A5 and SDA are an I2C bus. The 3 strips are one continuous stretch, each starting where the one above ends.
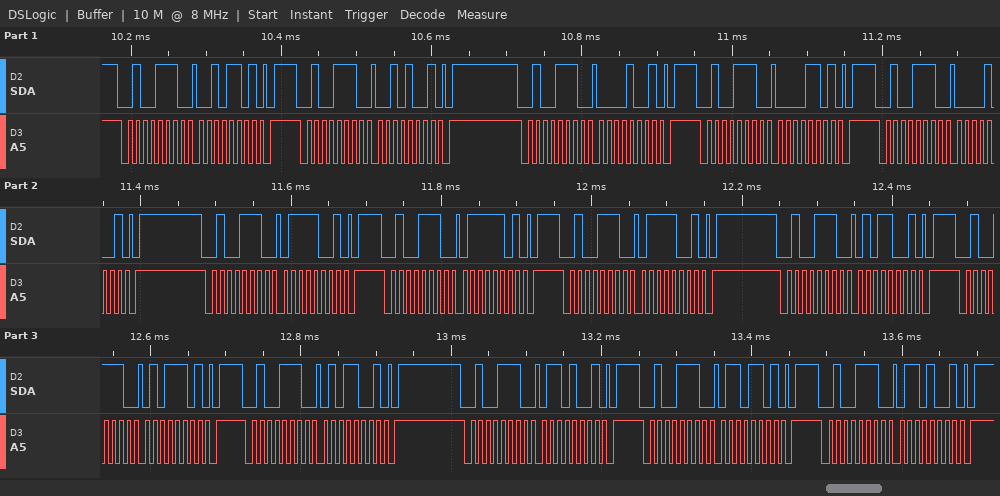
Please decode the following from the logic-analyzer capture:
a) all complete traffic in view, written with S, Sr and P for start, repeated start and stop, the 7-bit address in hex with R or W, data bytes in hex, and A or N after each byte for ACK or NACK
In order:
S 27W A 2D A P S 27W A 29 A P S 27W A 09 A P S 27W A 0D A P S 27W A 09 A P S 27W A 79 A P S 27W A 7D A P S 27W A 79 A P S 27W A 59 A P S 27W A 5D A P S 27W A 59 A P S 27W A 69 A P S 27W A 6D A P S 27W A 69 A P
